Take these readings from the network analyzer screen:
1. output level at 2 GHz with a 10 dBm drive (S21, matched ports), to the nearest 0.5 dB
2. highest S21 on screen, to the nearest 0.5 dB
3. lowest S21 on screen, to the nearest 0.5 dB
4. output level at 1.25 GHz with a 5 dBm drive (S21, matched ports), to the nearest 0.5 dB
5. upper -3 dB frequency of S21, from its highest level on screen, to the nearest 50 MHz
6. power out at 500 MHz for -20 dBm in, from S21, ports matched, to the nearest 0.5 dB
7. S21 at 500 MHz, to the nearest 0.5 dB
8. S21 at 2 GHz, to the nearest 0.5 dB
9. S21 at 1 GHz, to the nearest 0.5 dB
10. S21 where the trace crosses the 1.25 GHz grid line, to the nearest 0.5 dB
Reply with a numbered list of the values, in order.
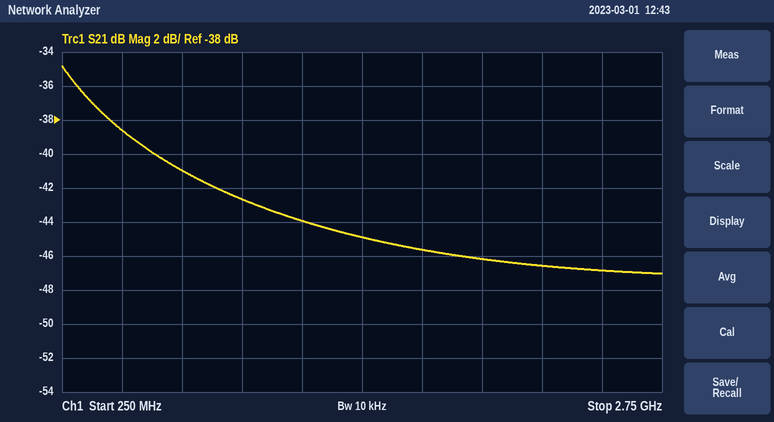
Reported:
1. -36.0 dBm
2. -35.0 dB
3. -47.0 dB
4. -39.0 dBm
5. 450 MHz
6. -58.5 dBm
7. -38.5 dB
8. -46.0 dB
9. -42.5 dB
10. -44.0 dB
